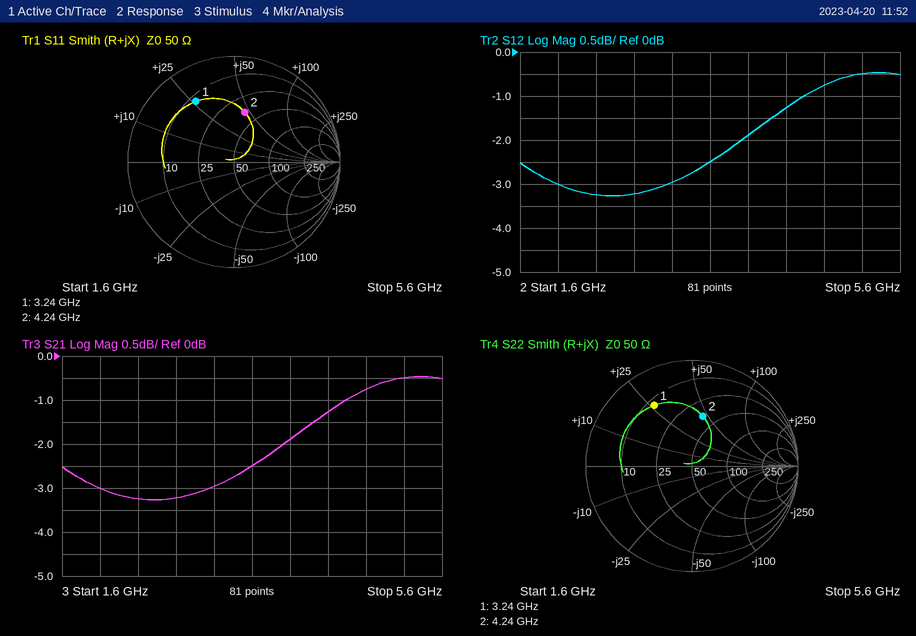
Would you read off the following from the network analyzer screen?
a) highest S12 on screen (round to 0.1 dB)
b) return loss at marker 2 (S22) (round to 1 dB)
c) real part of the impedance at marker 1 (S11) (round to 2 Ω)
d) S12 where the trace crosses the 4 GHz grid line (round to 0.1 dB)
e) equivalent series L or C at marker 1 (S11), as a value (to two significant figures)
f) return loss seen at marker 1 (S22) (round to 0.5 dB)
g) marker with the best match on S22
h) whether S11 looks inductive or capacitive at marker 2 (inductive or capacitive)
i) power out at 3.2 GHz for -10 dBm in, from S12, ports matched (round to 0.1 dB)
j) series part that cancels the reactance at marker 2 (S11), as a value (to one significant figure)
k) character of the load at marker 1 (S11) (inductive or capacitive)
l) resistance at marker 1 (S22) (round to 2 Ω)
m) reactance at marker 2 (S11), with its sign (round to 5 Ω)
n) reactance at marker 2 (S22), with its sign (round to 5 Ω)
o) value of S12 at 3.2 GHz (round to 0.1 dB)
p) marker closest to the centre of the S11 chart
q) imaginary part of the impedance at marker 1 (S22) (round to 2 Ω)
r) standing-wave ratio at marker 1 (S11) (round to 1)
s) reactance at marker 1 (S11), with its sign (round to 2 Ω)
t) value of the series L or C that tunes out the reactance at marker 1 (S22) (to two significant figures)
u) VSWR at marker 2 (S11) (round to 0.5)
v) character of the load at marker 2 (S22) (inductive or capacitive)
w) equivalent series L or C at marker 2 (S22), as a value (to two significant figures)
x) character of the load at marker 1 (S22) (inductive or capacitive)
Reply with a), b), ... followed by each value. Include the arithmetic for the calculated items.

a) -0.5 dB
b) 6 dB
c) 12 Ω
d) -1.9 dB
e) L = 26 Ω/(2π × 3.24 GHz) ≈ 1.3 nH
f) 3.5 dB
g) marker 2
h) inductive
i) -10 dBm + (-3.0 dB) = -13.0 dBm
j) C = 1/(2π × 4.24 GHz × 45 Ω) ≈ 834 fF, so 800 fF to one significant figure
k) inductive
l) 12 Ω
m) +45 Ω
n) +45 Ω
o) -3.0 dB
p) marker 2
q) +26 Ω
r) 5
s) +26 Ω
t) C = 1/(2π × 3.24 GHz × 26 Ω) ≈ 1.9 pF
u) 3.0
v) inductive
w) L = 45 Ω/(2π × 4.24 GHz) ≈ 1.7 nH
x) inductive
